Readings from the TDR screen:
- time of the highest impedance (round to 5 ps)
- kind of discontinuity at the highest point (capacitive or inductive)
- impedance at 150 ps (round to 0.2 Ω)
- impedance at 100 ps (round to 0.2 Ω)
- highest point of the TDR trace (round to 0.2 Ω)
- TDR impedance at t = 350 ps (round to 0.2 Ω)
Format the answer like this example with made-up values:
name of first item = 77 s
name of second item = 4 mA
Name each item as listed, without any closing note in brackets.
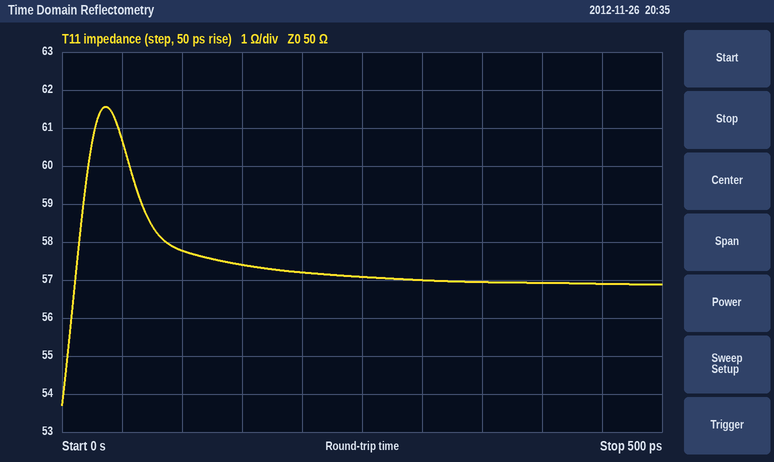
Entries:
time of the highest impedance = 35 ps
kind of discontinuity at the highest point = inductive
impedance at 150 ps = 57.4 Ω
impedance at 100 ps = 57.8 Ω
highest point of the TDR trace = 61.6 Ω
TDR impedance at t = 350 ps = 57.0 Ω
